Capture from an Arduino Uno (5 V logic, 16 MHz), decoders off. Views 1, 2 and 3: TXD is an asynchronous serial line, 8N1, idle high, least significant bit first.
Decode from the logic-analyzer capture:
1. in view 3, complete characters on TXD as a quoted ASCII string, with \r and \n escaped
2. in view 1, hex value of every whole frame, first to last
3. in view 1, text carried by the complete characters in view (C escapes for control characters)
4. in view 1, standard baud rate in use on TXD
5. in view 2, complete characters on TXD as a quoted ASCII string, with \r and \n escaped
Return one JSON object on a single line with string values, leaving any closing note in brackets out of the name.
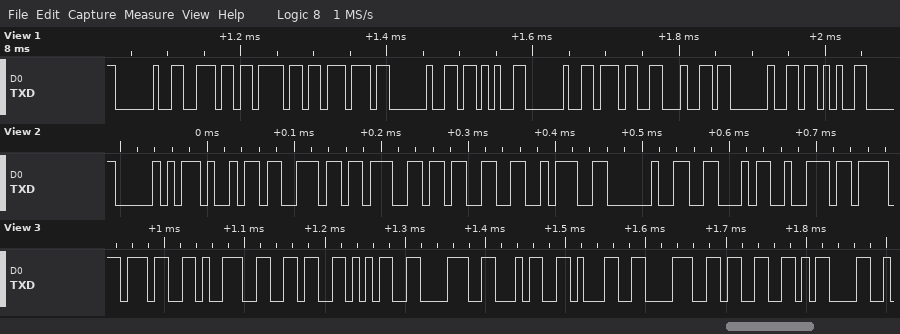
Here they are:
{"in view 3, complete characters on TXD as a quoted ASCII string, with \\r and \\n escaped": "\"796584183\\r\"", "in view 1, hex value of every whole frame, first to last": "20 6E 6F 77 20 2B 20 37 64 20 2B", "in view 1, text carried by the complete characters in view": "\" now + 7d +\"", "in view 1, standard baud rate in use on TXD": "115200 baud", "in view 2, complete characters on TXD as a quoted ASCII string, with \\r and \\n escaped": "\"Ping3: Fr\""}
